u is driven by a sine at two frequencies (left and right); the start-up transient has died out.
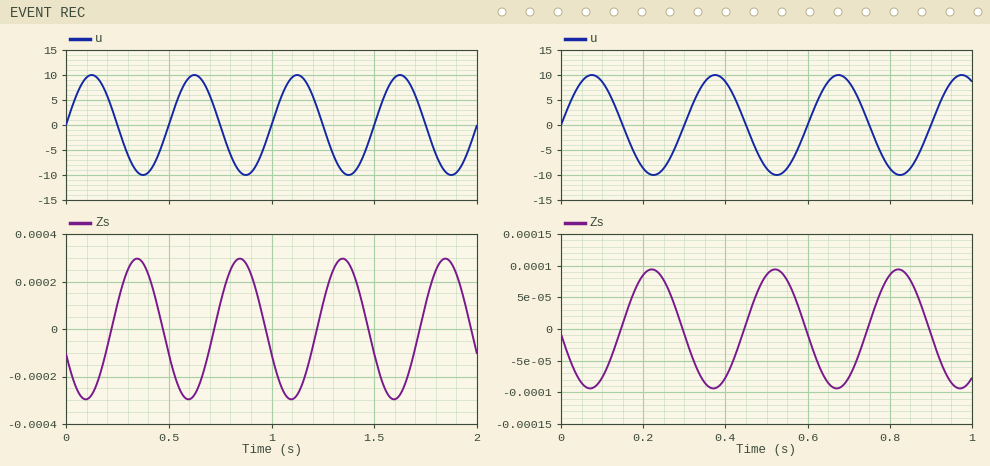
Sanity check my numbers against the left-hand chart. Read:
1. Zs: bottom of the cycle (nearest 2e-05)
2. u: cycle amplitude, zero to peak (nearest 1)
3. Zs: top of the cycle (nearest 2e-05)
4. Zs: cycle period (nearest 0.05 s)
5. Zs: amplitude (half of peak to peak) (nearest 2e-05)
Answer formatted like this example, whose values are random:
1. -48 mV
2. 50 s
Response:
1. -0.00030
2. 10
3. 0.00030
4. 0.50 s
5. 0.00030
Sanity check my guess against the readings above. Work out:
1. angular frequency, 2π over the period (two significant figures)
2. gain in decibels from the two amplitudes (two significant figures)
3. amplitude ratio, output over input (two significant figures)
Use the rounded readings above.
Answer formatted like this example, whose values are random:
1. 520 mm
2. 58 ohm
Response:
1. 13 rad/s
2. -90 dB
3. 0.000030
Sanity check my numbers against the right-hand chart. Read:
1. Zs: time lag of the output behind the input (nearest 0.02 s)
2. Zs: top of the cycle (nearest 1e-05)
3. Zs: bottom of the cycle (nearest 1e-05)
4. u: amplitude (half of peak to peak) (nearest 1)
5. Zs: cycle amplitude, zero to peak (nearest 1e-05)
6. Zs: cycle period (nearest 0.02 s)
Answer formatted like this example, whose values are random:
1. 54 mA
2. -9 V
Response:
1. 0.14 s
2. 0.00009
3. -0.00009
4. 10
5. 0.00009
6. 0.30 s
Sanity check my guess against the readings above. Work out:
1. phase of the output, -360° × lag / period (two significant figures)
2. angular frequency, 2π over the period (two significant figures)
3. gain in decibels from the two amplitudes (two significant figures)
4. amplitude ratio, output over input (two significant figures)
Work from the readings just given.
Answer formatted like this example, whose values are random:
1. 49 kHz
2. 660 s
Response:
1. -170°
2. 21 rad/s
3. -100 dB
4. 0.0000090
